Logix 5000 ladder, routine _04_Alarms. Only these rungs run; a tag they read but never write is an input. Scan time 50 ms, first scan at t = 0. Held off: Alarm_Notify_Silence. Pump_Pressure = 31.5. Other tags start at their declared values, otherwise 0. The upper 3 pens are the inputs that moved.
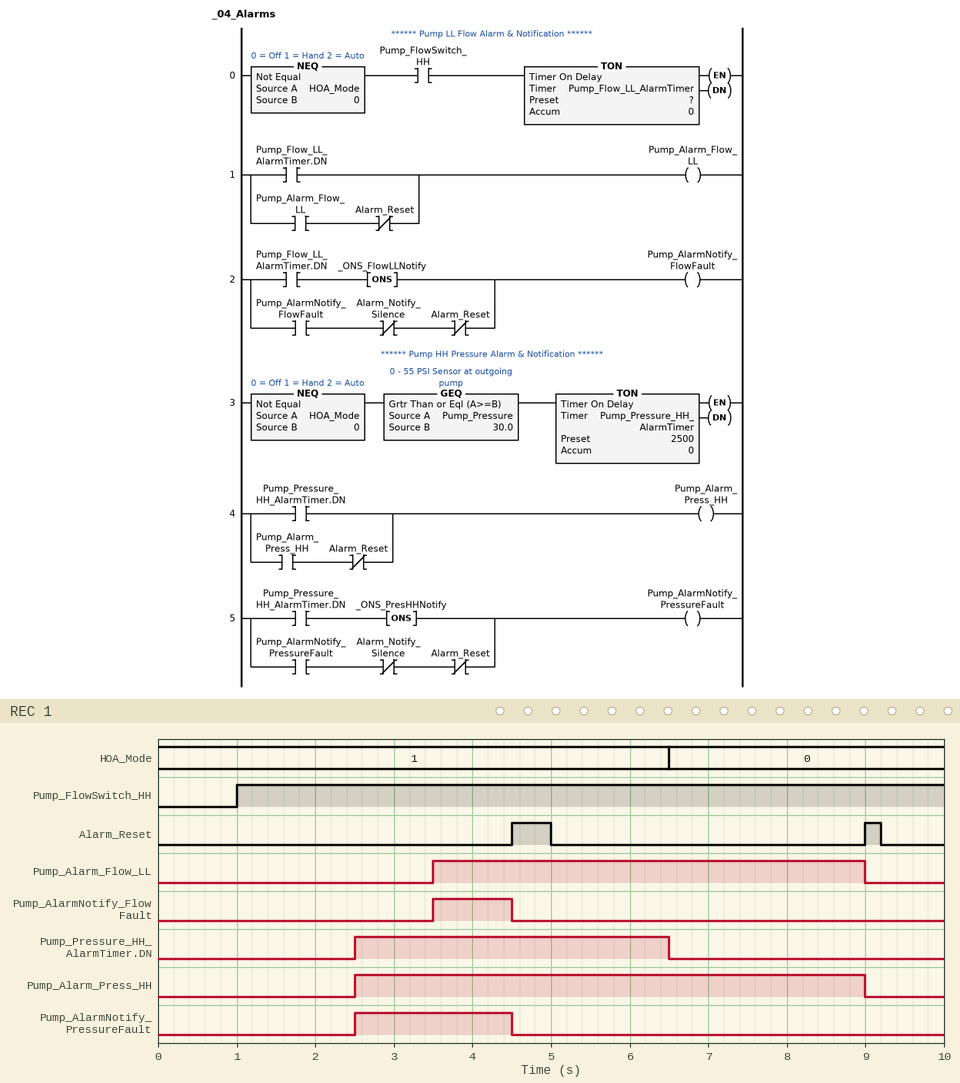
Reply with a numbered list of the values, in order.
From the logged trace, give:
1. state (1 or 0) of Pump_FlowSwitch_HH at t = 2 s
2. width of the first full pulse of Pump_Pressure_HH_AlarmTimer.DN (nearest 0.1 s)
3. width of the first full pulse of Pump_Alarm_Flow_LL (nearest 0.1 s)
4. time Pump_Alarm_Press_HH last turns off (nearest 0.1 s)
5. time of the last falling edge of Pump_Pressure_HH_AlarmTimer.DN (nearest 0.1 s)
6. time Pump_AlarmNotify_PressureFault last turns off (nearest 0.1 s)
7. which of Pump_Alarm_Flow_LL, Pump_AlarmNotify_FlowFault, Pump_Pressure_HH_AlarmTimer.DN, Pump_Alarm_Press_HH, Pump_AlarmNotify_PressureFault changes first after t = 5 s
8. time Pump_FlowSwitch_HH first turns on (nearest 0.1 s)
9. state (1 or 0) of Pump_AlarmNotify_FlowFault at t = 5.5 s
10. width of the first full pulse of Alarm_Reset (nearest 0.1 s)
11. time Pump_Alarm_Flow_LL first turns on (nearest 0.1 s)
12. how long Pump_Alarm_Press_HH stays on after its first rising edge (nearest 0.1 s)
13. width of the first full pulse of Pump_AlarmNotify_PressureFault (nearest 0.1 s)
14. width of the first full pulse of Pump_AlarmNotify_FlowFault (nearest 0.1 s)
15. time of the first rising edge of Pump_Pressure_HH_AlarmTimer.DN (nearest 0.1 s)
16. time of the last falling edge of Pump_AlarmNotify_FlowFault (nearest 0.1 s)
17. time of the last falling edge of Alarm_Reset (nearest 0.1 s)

1. 1
2. 4.0 s
3. 5.5 s
4. 9.0 s
5. 6.5 s
6. 4.5 s
7. Pump_Pressure_HH_AlarmTimer.DN
8. 1.0 s
9. 0
10. 0.5 s
11. 3.5 s
12. 6.5 s
13. 2.0 s
14. 1.0 s
15. 2.5 s
16. 4.5 s
17. 9.2 s
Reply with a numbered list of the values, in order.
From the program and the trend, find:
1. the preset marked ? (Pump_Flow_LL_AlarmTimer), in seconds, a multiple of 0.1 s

1. 2.5 s
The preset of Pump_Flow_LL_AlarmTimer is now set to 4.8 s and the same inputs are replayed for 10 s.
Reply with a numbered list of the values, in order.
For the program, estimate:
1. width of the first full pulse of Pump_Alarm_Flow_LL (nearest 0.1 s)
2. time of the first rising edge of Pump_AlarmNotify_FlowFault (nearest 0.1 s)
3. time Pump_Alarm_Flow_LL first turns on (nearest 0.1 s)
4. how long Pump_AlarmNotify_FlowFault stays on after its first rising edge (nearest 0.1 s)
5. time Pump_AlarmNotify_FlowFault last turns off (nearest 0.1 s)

1. 3.2 s
2. 5.8 s
3. 5.8 s
4. 3.2 s
5. 9.0 s
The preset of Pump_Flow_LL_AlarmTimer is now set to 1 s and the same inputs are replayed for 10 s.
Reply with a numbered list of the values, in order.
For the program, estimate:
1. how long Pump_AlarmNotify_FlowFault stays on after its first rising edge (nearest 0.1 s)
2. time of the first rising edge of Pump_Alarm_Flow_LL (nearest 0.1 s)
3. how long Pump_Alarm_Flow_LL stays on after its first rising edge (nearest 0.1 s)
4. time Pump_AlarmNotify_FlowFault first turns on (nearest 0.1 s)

1. 2.5 s
2. 2.0 s
3. 7.0 s
4. 2.0 s
